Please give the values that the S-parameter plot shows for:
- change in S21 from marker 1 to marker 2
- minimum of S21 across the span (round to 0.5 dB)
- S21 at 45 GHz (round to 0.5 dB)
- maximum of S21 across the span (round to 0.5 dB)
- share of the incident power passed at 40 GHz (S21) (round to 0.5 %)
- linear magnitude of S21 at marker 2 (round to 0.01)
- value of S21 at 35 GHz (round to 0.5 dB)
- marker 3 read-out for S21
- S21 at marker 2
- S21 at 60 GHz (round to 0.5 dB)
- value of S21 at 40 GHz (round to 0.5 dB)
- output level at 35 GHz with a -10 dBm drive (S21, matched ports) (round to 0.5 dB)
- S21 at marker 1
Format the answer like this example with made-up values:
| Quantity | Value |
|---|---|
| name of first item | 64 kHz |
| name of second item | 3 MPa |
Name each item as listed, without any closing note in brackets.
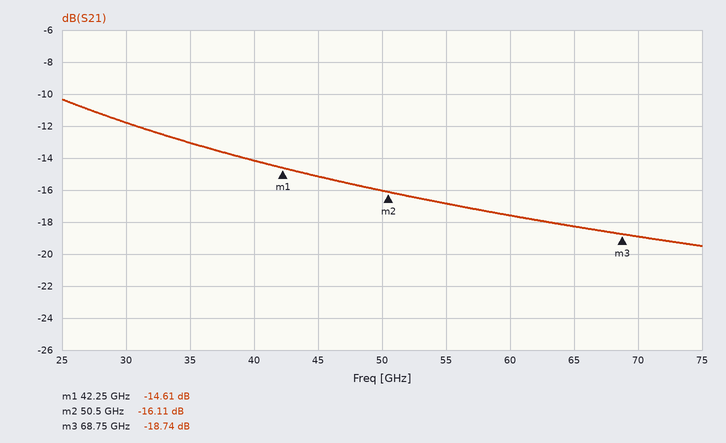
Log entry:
| Quantity | Value |
|---|---|
| change in S21 from marker 1 to marker 2 | -1.50 dB |
| minimum of S21 across the span | -19.5 dB |
| S21 at 45 GHz | -15.0 dB |
| maximum of S21 across the span | -10.5 dB |
| share of the incident power passed at 40 GHz (S21) | 4.0 % |
| linear magnitude of S21 at marker 2 | 0.16 |
| value of S21 at 35 GHz | -13.0 dB |
| marker 3 read-out for S21 | -18.74 dB |
| S21 at marker 2 | -16.11 dB |
| S21 at 60 GHz | -17.5 dB |
| value of S21 at 40 GHz | -14.0 dB |
| output level at 35 GHz with a -10 dBm drive (S21, matched ports) | -23.0 dBm |
| S21 at marker 1 | -14.61 dB |
